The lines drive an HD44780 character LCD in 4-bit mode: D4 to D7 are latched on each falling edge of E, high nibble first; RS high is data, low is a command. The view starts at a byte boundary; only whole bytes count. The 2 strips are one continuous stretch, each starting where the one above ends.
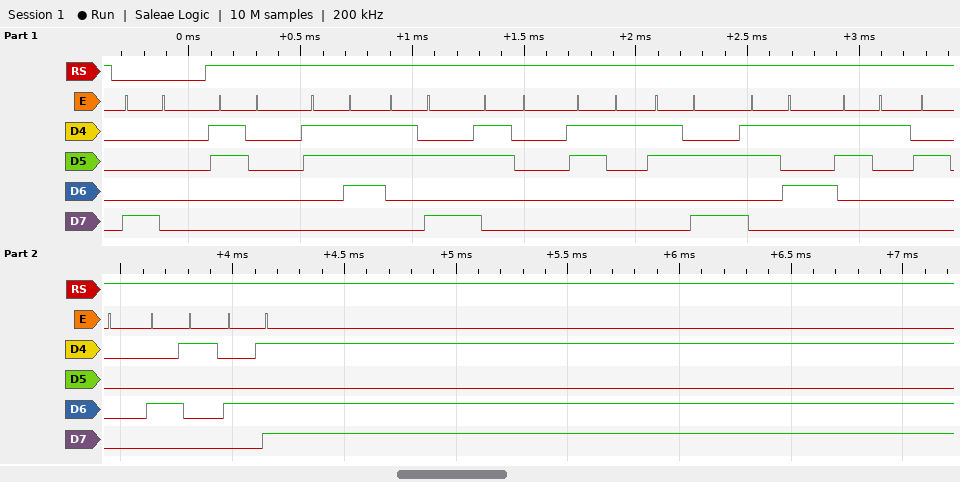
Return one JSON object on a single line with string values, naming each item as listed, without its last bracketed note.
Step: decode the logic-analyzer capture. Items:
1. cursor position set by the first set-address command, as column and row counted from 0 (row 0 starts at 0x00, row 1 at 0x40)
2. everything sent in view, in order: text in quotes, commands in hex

{"cursor position set by the first set-address command, as column and row counted from 0": "column 0, row 0", "everything sent in view, in order: text in quotes, commands in hex": "0x80 \"07:01:51 AM\""}
